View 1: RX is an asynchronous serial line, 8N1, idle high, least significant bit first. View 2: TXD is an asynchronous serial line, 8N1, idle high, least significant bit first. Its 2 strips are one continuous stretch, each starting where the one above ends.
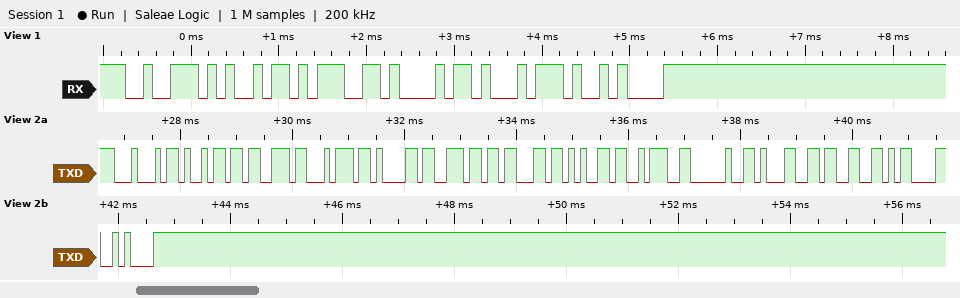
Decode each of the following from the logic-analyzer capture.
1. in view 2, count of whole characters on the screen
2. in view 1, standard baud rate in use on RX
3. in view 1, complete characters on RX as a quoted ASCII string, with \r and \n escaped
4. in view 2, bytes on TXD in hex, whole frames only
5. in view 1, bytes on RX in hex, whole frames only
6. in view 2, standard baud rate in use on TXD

14
9600 baud
"right\n"
44 69 73 74 61 6E 63 65 3A 20 31 33 0D 0A
0x72 0x69 0x67 0x68 0x74 0x0A
9600 baud
